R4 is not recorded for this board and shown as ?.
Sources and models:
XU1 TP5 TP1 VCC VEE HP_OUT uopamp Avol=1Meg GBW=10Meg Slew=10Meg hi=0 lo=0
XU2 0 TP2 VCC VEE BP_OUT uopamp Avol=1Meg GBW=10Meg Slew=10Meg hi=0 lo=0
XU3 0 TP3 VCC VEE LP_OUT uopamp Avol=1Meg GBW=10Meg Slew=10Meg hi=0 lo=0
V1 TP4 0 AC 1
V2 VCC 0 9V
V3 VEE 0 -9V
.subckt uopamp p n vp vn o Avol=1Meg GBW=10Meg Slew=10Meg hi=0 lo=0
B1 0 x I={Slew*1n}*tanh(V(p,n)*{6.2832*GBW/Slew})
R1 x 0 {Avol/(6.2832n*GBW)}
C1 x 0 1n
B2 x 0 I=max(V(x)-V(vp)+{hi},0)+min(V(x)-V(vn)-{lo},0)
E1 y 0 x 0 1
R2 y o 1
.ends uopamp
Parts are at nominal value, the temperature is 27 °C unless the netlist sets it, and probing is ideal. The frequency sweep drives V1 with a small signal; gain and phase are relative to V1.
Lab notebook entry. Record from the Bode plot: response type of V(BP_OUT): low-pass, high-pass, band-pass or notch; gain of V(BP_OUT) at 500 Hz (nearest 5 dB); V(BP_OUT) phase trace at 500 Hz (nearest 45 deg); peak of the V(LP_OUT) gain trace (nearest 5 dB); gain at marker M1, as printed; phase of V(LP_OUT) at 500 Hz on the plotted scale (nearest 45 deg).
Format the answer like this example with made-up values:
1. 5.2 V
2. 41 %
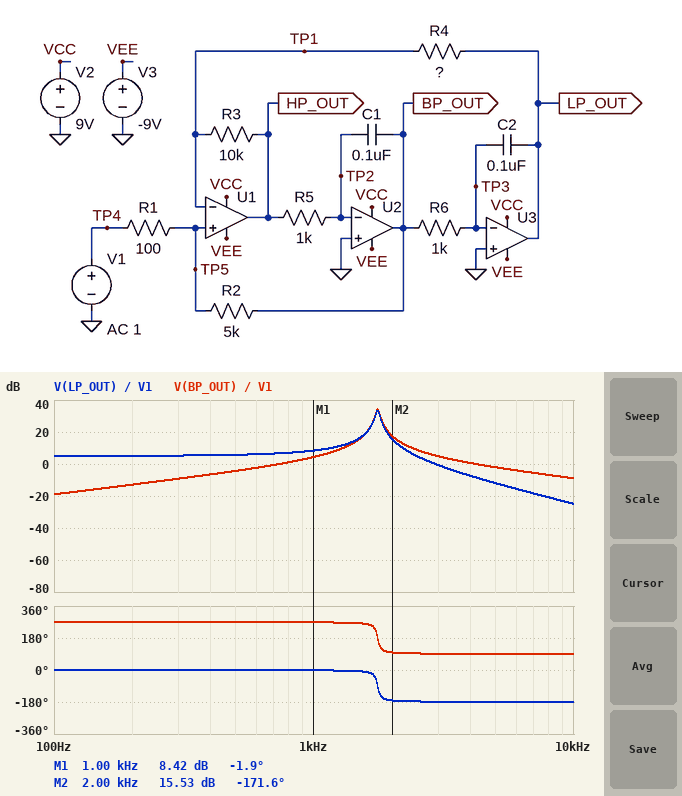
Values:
1. band-pass
2. -5 dB
3. 270 deg
4. 35 dB
5. 8.42 dB
6. 0 deg
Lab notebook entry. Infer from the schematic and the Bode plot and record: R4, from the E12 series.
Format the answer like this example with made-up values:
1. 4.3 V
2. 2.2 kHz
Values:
1. 8.2 kΩ
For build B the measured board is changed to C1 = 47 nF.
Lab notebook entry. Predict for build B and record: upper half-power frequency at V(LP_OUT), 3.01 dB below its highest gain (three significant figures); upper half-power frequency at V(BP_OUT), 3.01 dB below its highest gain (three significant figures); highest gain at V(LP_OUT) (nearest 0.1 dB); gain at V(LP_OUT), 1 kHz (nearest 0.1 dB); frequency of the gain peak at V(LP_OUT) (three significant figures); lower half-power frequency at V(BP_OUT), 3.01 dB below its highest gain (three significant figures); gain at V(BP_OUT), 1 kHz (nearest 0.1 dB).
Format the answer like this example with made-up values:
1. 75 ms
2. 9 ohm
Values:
1. 2.63 kHz
2. 2.64 kHz
3. 30.0 dB
4. 6.5 dB
5. 2.56 kHz
6. 2.49 kHz
7. 2.4 dB
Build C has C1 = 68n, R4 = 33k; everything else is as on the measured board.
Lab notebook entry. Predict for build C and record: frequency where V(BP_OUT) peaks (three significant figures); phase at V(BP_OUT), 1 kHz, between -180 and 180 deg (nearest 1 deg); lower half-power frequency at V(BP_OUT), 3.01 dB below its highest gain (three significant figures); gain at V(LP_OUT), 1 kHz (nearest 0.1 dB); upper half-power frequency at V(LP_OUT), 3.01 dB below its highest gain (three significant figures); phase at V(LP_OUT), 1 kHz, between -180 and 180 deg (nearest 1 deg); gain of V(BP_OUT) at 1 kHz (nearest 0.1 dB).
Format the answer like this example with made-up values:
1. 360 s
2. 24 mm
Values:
1. 1.06 kHz
2. -115 deg
3. 1.03 kHz
4. 30.5 dB
5. 1.09 kHz
6. -25 deg
7. 26.5 dB
